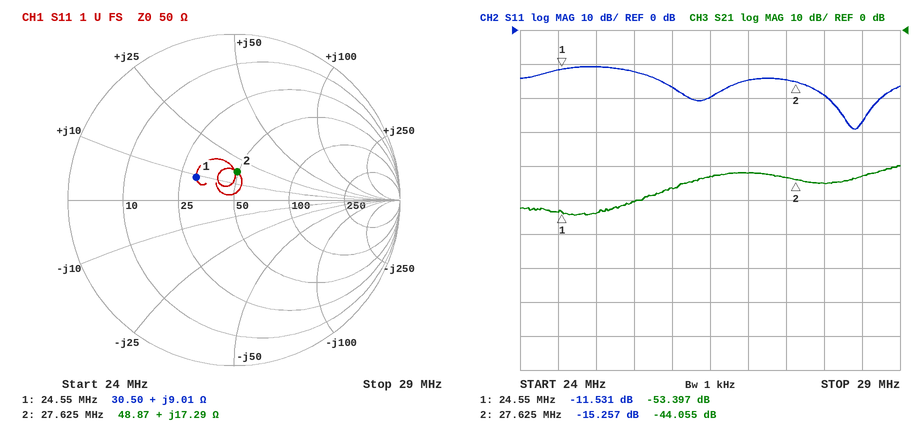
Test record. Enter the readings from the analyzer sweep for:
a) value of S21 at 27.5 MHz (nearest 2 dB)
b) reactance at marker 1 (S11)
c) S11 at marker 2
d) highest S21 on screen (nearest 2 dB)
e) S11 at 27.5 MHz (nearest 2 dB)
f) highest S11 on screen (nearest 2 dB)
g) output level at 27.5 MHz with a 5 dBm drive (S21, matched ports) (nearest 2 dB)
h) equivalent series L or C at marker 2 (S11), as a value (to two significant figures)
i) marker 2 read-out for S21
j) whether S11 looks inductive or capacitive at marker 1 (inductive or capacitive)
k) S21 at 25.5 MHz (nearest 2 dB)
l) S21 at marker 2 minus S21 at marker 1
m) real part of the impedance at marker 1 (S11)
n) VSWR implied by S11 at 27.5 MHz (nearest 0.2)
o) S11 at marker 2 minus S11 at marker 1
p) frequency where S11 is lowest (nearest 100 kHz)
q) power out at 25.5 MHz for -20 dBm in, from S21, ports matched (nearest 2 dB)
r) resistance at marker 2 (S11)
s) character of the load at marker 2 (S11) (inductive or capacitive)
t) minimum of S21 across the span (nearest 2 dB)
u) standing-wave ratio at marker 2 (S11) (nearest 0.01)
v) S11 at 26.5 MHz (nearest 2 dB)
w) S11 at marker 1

-44 dB
+9.01 Ω
-15.257 dB
-40 dB
-14 dB
-10 dB
-38 dBm
100 nH
-44.055 dB
inductive
-50 dB
9.342 dB
30.50 Ω
1.4
-3.726 dB
28.4 MHz
-70 dBm
48.87 Ω
inductive
-54 dB
1.42
-20 dB
-11.531 dB
